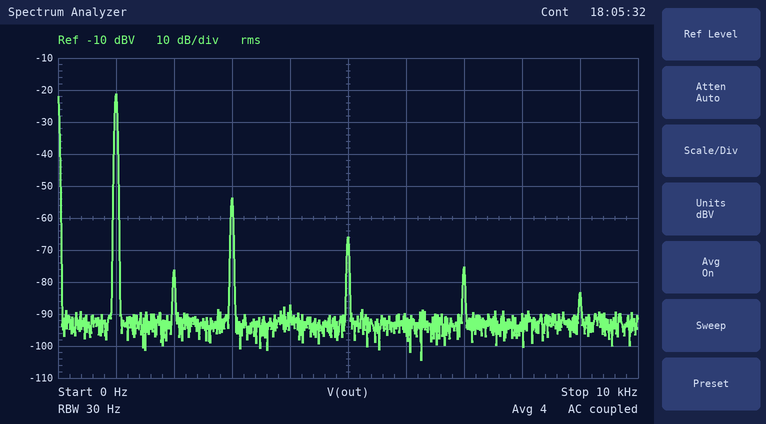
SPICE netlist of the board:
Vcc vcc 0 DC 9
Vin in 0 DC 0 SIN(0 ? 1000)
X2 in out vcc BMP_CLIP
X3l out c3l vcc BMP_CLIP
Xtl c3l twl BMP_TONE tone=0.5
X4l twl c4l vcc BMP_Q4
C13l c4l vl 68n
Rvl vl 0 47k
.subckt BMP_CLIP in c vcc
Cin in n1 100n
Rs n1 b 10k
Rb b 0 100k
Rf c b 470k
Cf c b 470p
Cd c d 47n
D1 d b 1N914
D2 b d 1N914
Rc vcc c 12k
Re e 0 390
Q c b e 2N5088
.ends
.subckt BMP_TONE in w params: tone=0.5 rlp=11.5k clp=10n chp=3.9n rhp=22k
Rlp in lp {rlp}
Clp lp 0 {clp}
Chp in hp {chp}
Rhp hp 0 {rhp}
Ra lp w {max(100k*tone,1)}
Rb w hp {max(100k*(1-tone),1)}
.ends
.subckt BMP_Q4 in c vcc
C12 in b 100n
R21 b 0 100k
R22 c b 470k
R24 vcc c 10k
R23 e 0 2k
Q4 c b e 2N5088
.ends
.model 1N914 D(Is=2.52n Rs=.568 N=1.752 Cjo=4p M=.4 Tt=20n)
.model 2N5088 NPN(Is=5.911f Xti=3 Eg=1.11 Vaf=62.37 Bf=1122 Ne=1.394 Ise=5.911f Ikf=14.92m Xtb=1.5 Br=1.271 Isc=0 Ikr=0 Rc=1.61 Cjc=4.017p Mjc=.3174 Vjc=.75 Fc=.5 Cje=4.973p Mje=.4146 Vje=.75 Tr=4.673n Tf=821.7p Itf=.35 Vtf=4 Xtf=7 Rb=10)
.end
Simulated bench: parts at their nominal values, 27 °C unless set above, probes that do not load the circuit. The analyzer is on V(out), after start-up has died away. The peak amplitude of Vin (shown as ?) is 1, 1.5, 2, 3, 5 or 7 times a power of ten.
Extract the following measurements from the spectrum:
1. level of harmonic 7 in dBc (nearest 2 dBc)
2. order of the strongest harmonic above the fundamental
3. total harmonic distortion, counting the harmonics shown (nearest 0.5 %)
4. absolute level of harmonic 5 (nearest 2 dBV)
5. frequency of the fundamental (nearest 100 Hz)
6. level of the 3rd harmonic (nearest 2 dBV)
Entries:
-54 dBc
3
2.5 %
-66 dBV
1.0 kHz
-54 dBV
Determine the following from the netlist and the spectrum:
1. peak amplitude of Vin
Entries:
15 mV
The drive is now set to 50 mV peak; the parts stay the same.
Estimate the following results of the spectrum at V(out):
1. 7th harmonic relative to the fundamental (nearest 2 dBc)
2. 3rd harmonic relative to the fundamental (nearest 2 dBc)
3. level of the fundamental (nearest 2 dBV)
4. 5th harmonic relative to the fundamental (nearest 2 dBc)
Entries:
-46 dBc
-20 dBc
-14 dBV
-36 dBc
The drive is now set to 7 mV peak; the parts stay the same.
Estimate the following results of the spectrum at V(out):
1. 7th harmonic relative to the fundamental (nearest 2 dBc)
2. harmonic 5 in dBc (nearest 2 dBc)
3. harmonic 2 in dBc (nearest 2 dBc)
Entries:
-60 dBc
-48 dBc
-58 dBc
